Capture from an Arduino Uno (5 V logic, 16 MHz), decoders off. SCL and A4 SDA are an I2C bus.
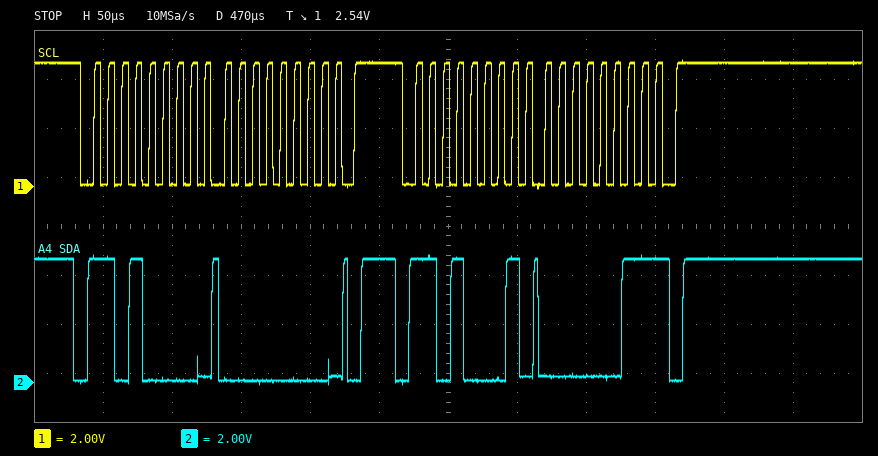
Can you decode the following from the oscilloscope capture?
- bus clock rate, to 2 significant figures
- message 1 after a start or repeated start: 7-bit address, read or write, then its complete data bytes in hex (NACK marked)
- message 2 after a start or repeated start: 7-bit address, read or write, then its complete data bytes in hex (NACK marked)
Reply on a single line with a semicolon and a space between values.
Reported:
100 kHz; 0x68 write: 00; 0x68 read: 03 NACK
